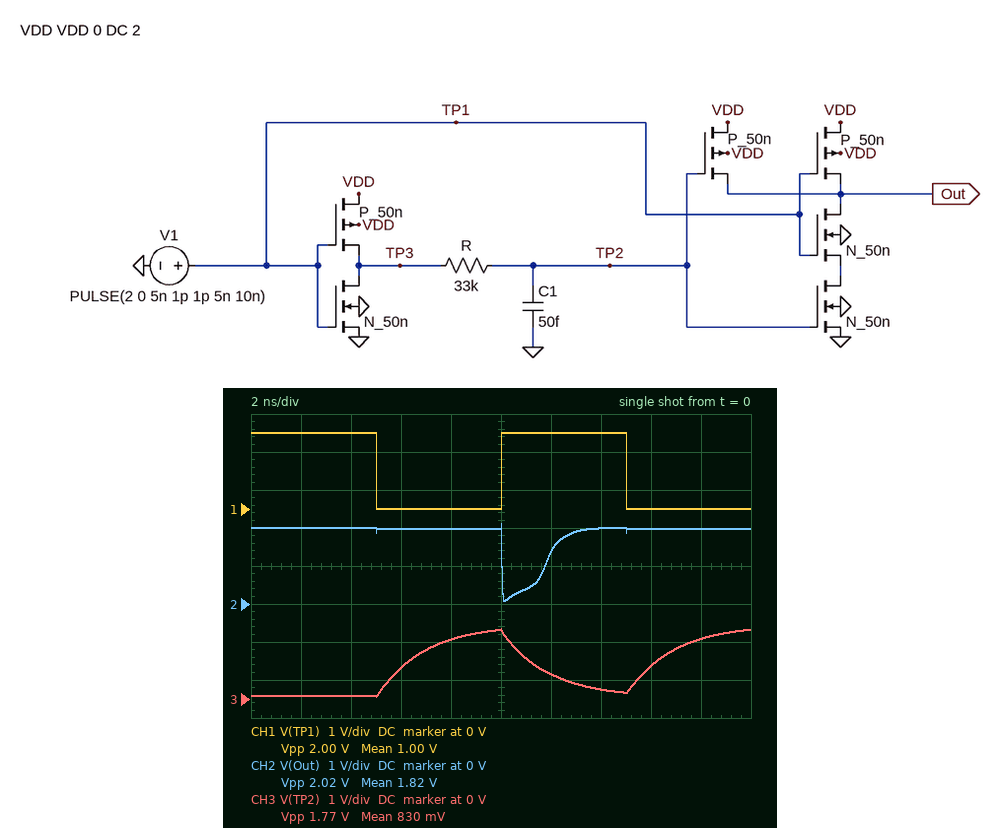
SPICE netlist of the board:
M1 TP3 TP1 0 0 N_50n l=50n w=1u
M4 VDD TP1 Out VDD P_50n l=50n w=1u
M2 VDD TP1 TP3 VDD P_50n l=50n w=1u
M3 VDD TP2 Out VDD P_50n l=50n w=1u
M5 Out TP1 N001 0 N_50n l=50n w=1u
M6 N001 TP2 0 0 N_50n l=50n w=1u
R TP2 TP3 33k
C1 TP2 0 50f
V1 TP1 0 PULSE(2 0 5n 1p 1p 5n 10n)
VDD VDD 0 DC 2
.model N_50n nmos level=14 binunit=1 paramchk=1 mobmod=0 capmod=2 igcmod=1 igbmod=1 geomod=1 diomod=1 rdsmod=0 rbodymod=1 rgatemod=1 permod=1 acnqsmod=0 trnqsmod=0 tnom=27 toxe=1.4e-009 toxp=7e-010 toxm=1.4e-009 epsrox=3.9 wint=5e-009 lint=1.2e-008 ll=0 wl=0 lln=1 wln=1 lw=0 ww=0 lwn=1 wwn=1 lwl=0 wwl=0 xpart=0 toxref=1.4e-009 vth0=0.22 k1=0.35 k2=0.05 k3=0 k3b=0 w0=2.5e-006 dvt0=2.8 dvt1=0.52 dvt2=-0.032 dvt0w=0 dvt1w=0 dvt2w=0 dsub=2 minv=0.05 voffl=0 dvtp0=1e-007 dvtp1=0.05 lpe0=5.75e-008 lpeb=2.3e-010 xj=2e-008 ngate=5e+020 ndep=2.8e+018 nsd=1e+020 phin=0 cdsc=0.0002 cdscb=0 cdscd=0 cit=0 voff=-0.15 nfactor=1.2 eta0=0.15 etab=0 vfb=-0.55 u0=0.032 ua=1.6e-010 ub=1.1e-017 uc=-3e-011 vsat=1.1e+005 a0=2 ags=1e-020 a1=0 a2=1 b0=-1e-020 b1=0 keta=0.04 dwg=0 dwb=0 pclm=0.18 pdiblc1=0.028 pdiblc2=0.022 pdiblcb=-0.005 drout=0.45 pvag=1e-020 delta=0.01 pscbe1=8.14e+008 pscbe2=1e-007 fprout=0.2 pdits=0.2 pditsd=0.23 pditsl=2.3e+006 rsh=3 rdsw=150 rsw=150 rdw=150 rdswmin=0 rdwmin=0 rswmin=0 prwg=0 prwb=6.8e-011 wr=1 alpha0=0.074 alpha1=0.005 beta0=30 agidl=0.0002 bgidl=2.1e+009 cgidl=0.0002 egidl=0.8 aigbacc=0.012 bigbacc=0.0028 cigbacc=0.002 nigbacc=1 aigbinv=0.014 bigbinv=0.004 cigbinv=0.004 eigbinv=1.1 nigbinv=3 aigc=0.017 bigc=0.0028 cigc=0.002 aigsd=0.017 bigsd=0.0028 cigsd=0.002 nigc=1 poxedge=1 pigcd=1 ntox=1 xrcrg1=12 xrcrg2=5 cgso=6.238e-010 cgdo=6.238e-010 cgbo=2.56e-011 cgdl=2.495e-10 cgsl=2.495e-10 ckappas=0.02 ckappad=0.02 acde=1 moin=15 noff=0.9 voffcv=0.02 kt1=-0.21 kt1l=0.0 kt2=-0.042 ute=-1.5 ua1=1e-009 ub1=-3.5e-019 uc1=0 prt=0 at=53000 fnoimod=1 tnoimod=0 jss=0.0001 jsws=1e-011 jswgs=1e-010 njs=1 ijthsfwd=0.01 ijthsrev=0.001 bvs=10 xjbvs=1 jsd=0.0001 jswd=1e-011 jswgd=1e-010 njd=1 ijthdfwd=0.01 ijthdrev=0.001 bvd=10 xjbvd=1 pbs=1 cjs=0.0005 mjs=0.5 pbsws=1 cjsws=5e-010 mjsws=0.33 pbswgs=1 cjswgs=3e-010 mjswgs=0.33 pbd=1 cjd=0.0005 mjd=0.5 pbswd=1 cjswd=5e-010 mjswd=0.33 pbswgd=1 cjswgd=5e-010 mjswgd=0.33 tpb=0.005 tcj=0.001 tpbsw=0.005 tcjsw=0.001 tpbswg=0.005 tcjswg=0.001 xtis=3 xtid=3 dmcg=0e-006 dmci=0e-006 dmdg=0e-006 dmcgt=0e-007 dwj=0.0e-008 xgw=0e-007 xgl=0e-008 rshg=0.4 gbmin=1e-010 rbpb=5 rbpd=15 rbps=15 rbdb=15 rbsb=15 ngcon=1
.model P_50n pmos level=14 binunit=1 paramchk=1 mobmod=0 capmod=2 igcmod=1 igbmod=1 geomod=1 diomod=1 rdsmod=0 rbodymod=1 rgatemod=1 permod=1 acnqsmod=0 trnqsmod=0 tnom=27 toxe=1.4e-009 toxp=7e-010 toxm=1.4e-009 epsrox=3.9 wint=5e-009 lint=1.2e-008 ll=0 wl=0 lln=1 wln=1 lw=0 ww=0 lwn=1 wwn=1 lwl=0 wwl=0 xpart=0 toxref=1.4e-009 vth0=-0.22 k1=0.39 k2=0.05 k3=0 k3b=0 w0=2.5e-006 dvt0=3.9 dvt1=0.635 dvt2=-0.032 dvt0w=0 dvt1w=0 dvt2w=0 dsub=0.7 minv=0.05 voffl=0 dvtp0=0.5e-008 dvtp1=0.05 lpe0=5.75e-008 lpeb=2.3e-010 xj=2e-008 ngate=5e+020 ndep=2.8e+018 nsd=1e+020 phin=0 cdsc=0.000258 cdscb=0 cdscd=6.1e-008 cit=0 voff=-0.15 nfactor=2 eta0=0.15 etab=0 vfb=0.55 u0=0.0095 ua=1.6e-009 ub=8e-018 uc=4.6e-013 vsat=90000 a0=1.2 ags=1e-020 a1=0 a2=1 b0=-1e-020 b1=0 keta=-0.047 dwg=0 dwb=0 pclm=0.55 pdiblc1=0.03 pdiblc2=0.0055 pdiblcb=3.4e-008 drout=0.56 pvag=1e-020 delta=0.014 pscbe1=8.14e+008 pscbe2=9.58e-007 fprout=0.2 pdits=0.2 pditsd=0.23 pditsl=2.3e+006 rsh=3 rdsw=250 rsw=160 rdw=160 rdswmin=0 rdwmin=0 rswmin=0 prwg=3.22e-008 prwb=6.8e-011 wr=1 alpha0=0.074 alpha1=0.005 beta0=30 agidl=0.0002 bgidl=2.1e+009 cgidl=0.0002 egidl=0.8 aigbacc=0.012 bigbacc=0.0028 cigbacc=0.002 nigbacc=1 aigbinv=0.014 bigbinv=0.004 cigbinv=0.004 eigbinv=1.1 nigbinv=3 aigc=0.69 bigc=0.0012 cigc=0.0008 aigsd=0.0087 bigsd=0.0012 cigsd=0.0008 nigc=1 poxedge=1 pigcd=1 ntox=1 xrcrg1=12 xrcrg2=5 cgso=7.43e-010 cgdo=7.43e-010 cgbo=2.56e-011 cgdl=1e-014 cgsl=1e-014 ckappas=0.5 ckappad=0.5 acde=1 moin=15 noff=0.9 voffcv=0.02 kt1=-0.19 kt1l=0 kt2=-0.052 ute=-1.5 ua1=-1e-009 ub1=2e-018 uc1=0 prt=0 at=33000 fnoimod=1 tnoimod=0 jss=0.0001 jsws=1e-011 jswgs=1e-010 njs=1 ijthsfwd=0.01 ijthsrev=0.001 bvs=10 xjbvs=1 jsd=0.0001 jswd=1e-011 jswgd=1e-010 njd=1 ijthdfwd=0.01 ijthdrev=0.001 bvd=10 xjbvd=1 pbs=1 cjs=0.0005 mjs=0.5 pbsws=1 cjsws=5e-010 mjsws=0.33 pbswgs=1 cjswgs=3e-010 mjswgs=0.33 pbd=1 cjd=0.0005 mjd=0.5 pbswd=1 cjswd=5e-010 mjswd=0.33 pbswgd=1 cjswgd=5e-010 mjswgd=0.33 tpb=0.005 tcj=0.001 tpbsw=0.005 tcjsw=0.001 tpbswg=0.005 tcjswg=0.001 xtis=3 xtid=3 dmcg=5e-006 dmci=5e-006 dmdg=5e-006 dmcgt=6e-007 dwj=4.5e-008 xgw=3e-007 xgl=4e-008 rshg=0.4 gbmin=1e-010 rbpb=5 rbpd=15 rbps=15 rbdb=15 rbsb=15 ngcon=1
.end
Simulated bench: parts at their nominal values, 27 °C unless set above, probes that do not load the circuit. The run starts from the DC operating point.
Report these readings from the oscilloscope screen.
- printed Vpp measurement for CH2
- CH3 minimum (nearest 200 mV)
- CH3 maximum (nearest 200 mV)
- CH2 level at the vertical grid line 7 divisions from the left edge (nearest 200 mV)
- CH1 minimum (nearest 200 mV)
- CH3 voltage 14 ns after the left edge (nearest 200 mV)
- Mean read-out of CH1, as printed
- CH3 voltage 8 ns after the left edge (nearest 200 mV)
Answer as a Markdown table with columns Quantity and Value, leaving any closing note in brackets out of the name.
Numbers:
| Quantity | Value |
|---|---|
| printed Vpp measurement for CH2 | 2.02 V |
| CH3 minimum | 0 V |
| CH3 maximum | 1.8 V |
| CH2 level at the vertical grid line 7 divisions from the left edge | 2.0 V |
| CH1 minimum | 0 V |
| CH3 voltage 14 ns after the left edge | 200 mV |
| Mean read-out of CH1, as printed | 1.00 V |
| CH3 voltage 8 ns after the left edge | 1.6 V |
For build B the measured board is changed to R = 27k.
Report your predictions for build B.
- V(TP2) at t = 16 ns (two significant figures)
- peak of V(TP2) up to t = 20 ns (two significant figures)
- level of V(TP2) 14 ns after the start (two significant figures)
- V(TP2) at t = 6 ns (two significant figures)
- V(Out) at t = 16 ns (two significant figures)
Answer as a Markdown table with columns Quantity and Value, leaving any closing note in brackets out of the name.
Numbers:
| Quantity | Value |
|---|---|
| V(TP2) at t = 16 ns | 960 mV |
| peak of V(TP2) up to t = 20 ns | 1.9 V |
| level of V(TP2) 14 ns after the start | 170 mV |
| V(TP2) at t = 6 ns | 930 mV |
| V(Out) at t = 16 ns | 2.0 V |
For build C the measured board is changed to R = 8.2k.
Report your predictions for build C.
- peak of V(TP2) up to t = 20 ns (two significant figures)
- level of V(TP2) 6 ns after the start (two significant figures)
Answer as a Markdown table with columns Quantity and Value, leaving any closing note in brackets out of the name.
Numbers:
| Quantity | Value |
|---|---|
| peak of V(TP2) up to t = 20 ns | 2.0 V |
| level of V(TP2) 6 ns after the start | 1.7 V |
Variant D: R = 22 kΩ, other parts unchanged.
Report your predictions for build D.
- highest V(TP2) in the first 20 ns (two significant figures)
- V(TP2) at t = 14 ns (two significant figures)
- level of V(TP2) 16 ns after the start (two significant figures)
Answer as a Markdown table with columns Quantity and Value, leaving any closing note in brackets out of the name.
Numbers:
| Quantity | Value |
|---|---|
| highest V(TP2) in the first 20 ns | 1.9 V |
| V(TP2) at t = 14 ns | 120 mV |
| level of V(TP2) 16 ns after the start | 1.1 V |
